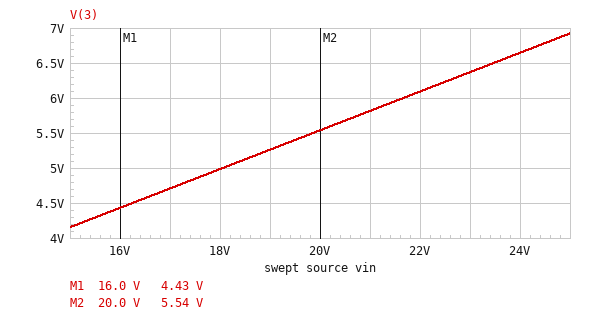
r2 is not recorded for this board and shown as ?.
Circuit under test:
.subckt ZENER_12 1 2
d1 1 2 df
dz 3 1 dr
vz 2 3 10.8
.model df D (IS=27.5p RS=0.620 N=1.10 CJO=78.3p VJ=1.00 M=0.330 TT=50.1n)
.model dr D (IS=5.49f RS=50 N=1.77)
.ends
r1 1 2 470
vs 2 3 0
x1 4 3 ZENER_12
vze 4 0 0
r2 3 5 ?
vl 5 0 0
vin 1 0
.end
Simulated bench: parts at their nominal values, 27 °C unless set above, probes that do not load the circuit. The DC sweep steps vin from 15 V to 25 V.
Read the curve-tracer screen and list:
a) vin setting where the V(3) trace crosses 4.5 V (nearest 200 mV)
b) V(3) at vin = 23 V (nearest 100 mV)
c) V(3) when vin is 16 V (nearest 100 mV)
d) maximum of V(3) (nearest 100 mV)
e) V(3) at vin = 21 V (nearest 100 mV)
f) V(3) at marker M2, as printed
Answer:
16.2 V
6.4 V
4.4 V
6.9 V
5.8 V
5.54 V
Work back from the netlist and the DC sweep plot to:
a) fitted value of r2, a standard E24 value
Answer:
180 Ω
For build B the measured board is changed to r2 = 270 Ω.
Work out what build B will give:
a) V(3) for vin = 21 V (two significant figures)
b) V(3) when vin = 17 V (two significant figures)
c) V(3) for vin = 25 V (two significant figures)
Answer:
7.7 V
6.2 V
9.1 V
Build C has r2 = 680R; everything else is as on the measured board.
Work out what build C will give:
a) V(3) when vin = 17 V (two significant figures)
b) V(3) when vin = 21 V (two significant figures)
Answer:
10 V
12 V
